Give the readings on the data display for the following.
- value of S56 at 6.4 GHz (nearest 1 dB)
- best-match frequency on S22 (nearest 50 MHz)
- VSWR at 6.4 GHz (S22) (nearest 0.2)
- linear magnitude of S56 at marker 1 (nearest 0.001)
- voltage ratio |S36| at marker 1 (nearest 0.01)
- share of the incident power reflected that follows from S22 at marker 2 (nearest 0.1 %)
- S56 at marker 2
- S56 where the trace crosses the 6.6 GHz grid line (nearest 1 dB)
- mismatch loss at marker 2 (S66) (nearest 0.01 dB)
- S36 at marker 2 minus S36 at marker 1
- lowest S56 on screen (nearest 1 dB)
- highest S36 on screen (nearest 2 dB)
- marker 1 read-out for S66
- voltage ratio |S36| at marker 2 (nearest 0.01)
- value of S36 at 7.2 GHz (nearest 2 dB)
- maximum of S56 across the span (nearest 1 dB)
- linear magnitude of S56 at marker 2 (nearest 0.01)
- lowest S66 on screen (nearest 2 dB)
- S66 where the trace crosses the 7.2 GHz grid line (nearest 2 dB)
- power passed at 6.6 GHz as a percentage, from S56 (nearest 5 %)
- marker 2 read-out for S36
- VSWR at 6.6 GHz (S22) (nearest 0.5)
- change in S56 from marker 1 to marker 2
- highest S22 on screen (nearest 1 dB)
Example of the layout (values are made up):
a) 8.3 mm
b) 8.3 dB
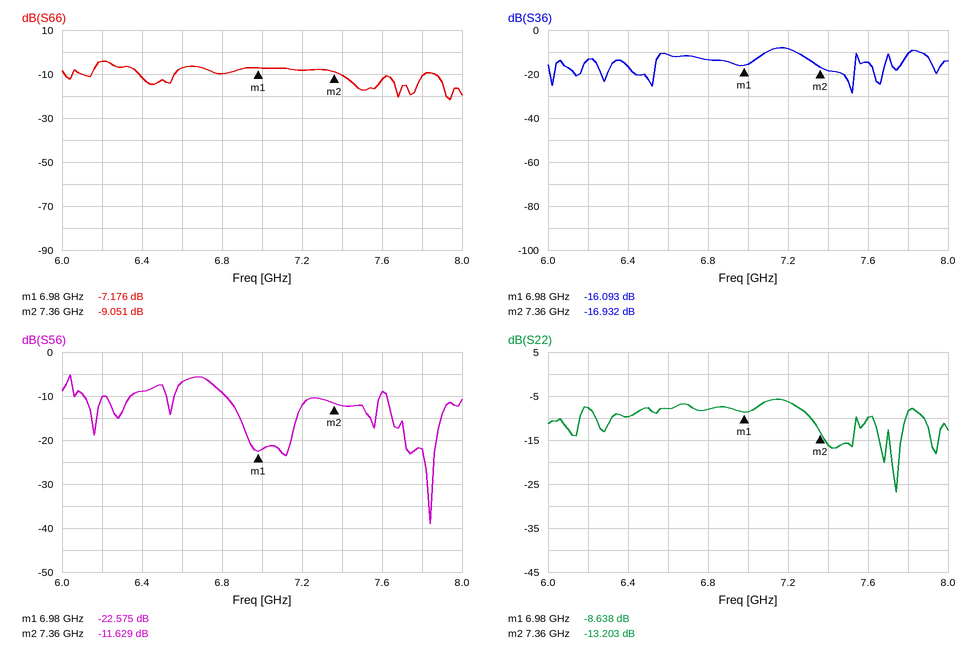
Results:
a) -9 dB
b) 7.75 GHz
c) 2.0
d) 0.074
e) 0.16
f) 4.8 %
g) -11.629 dB
h) -7 dB
i) 0.58 dB
j) -0.839 dB
k) -39 dB
l) -8 dB
m) -7.176 dB
n) 0.14
o) -8 dB
p) -5 dB
q) 0.26
r) -22 dB
s) -8 dB
t) 20 %
u) -16.932 dB
v) 2.5
w) 10.946 dB
x) -6 dB
